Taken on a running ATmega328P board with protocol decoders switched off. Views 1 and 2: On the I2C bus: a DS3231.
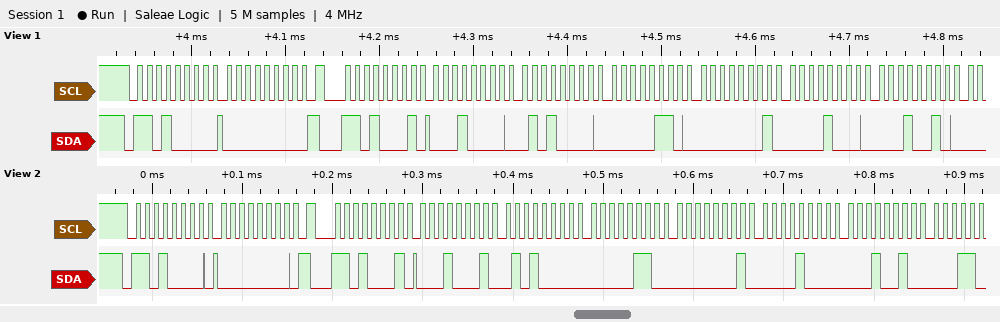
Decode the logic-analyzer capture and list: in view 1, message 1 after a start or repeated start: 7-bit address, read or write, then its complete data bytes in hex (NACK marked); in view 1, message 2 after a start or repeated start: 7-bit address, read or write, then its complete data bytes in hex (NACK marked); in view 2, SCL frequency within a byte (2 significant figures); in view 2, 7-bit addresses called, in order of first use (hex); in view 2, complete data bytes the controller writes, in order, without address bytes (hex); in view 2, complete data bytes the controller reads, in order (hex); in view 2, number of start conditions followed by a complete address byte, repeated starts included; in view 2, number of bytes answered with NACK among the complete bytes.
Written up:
0x68 write: 00
0x68 read: 10 50 06 01 08 12
100 kHz
0x68
00
11 50 06 01 08 12
2
0
